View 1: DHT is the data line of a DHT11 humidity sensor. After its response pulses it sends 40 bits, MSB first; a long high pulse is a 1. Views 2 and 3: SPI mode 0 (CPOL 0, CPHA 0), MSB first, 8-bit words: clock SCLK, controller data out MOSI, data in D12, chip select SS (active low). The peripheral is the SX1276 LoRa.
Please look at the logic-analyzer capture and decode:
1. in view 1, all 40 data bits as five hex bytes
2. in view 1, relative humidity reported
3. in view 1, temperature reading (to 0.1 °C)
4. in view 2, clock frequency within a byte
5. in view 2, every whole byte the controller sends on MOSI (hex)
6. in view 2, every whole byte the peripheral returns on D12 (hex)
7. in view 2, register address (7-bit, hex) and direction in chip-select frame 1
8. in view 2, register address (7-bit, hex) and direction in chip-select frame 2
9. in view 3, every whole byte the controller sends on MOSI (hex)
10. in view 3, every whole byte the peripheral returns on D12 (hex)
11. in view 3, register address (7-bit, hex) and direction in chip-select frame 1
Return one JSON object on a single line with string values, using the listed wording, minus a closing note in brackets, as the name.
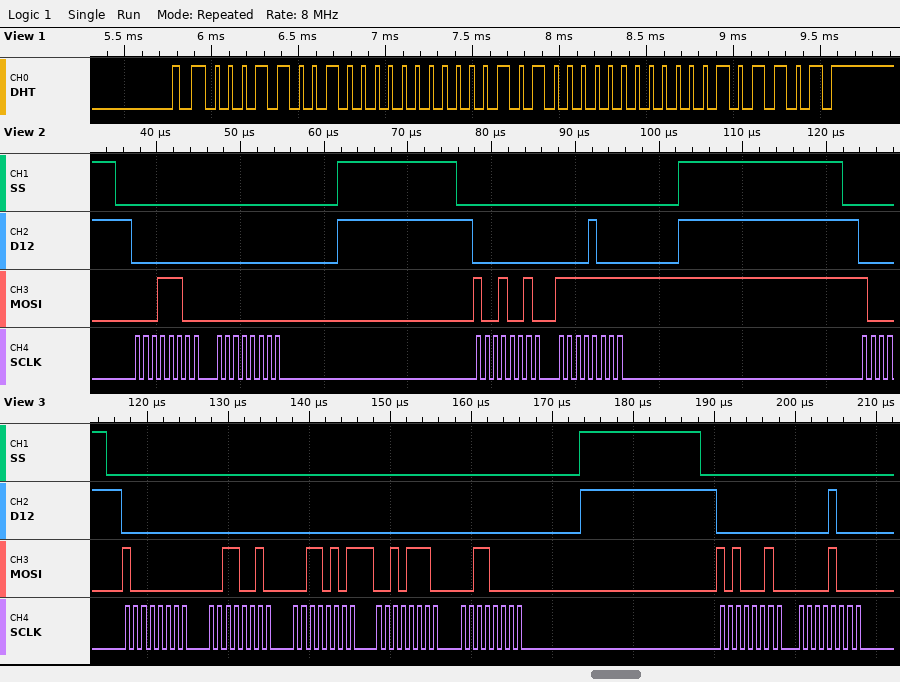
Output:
{"in view 1, all 40 data bits as five hex bytes": "19 00 14 00 2D", "in view 1, relative humidity reported": "25 %", "in view 1, temperature reading": "20.0 °C", "in view 2, clock frequency within a byte": "1 MHz", "in view 2, every whole byte the controller sends on MOSI": "1C 00 92 FF", "in view 2, every whole byte the peripheral returns on D12": "00 00 00 08", "in view 2, register address (7-bit, hex) and direction in chip-select frame 1": "0x1C read", "in view 2, register address (7-bit, hex) and direction in chip-select frame 2": "0x12 write", "in view 3, every whole byte the controller sends on MOSI": "80 32 35 2E 30 A2 08", "in view 3, every whole byte the peripheral returns on D12": "00 00 00 00 00 00 08", "in view 3, register address (7-bit, hex) and direction in chip-select frame 1": "0x00 write"}
